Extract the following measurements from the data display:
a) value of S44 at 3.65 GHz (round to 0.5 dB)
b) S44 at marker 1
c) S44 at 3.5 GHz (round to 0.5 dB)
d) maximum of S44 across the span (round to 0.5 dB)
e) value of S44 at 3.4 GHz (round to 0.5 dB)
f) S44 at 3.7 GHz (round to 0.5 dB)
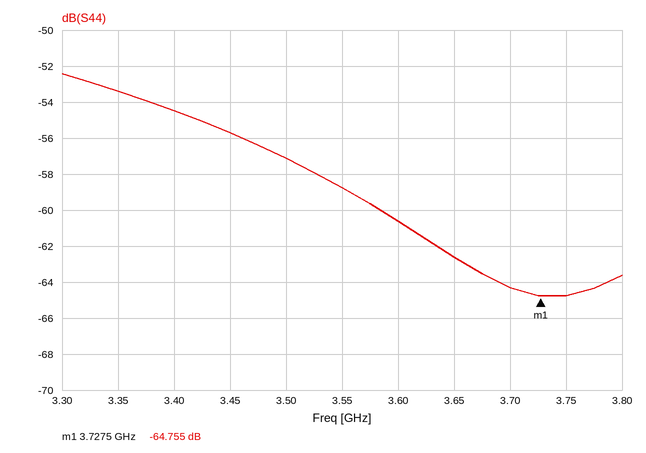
-62.5 dB
-64.755 dB
-57.0 dB
-52.5 dB
-54.5 dB
-64.5 dB
